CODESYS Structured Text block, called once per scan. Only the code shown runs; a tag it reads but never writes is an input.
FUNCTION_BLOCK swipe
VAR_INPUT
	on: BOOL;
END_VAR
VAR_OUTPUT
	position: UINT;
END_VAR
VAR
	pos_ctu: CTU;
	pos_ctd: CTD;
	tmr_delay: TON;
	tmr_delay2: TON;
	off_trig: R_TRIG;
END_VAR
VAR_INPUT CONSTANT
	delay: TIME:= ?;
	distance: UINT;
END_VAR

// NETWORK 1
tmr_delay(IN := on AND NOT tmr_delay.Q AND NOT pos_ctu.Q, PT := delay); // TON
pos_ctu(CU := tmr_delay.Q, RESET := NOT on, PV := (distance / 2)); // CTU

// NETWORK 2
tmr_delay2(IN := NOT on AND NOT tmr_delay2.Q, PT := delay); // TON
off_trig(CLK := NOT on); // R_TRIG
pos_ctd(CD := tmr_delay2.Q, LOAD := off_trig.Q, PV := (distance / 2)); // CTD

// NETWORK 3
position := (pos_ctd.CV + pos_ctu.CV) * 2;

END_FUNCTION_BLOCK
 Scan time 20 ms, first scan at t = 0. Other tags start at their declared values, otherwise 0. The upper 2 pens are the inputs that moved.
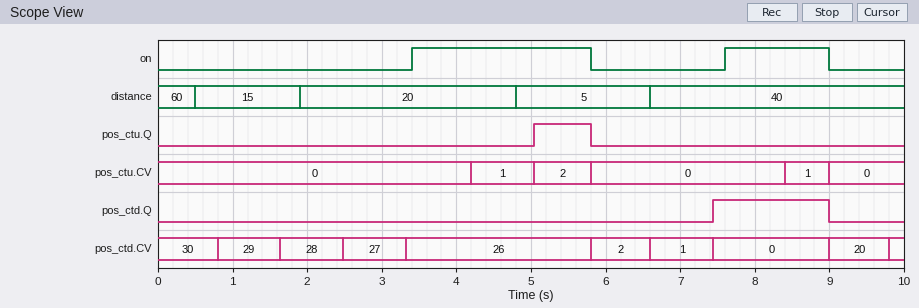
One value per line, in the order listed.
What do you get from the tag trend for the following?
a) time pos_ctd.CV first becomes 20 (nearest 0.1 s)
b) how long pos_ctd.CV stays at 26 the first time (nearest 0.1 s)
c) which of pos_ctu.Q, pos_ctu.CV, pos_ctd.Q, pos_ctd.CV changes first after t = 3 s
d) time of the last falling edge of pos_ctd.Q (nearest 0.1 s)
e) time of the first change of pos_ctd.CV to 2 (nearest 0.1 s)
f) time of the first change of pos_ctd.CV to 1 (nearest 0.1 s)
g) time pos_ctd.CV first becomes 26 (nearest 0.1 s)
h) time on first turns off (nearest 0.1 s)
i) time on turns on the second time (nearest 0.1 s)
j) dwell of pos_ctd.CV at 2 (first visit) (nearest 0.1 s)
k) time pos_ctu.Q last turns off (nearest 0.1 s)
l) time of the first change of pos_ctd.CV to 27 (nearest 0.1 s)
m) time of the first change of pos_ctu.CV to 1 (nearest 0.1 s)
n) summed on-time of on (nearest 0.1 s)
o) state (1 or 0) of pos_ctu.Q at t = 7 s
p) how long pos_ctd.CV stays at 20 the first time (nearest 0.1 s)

9.0 s
2.5 s
pos_ctd.CV
9.0 s
5.8 s
6.6 s
3.3 s
5.8 s
7.6 s
0.8 s
5.8 s
2.5 s
4.2 s
3.8 s
0
0.8 s
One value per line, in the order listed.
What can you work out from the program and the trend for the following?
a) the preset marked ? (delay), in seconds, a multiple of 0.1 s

0.8 s
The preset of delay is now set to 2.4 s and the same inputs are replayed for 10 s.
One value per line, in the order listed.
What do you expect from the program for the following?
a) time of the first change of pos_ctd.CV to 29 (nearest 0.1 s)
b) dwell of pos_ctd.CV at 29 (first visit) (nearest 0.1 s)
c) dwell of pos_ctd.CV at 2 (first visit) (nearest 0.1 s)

2.4 s
3.4 s
3.2 s
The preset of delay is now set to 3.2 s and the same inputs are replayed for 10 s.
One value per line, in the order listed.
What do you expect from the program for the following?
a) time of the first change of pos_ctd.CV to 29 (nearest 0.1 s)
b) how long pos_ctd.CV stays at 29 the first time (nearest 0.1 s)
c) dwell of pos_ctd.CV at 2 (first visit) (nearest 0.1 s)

3.2 s
2.6 s
3.2 s
